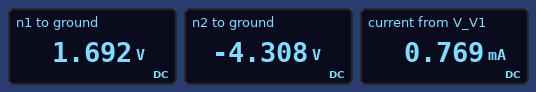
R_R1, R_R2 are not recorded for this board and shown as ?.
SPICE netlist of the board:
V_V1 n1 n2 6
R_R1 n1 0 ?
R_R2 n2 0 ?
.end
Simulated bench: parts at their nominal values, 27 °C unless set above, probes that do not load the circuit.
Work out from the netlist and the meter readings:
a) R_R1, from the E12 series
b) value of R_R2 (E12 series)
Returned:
2.2 kΩ
5.6 kΩ
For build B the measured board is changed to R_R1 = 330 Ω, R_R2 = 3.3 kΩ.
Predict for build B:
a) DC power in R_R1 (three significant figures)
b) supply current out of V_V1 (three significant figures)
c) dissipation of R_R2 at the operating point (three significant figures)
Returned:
902 µW
1.65 mA
9.02 mW
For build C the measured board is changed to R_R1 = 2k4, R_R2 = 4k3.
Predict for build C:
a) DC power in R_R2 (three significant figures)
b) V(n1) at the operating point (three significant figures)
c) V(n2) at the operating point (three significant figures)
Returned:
3.45 mW
2.15 V
-3.85 V
